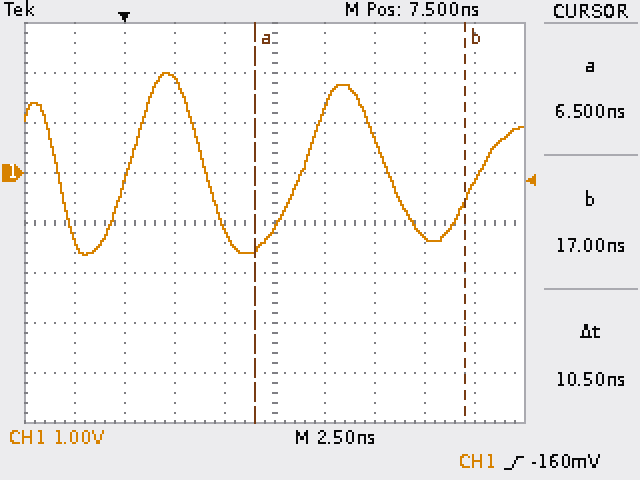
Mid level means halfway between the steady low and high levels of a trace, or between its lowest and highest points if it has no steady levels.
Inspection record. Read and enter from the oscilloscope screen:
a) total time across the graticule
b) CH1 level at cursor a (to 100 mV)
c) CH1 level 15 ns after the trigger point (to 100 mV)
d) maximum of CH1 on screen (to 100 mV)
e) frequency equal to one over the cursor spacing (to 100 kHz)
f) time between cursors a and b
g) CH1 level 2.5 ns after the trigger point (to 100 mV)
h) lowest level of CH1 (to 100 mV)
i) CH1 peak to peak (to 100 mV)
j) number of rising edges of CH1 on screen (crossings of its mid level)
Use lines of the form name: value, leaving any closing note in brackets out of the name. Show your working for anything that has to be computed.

total time across the graticule: 25 ns
CH1 level at cursor a: -1.5 V
CH1 level 15 ns after the trigger point: -1.3 V
maximum of CH1 on screen: 2.0 V
frequency equal to one over the cursor spacing: 1 / 10.5 ns ≈ 95.2 MHz
time between cursors a and b: 10.5 ns
CH1 level 2.5 ns after the trigger point: 1.9 V
lowest level of CH1: -1.6 V
CH1 peak to peak: 2.0 V − (-1.6 V) = 3.6 V
number of rising edges of CH1 on screen: 3
